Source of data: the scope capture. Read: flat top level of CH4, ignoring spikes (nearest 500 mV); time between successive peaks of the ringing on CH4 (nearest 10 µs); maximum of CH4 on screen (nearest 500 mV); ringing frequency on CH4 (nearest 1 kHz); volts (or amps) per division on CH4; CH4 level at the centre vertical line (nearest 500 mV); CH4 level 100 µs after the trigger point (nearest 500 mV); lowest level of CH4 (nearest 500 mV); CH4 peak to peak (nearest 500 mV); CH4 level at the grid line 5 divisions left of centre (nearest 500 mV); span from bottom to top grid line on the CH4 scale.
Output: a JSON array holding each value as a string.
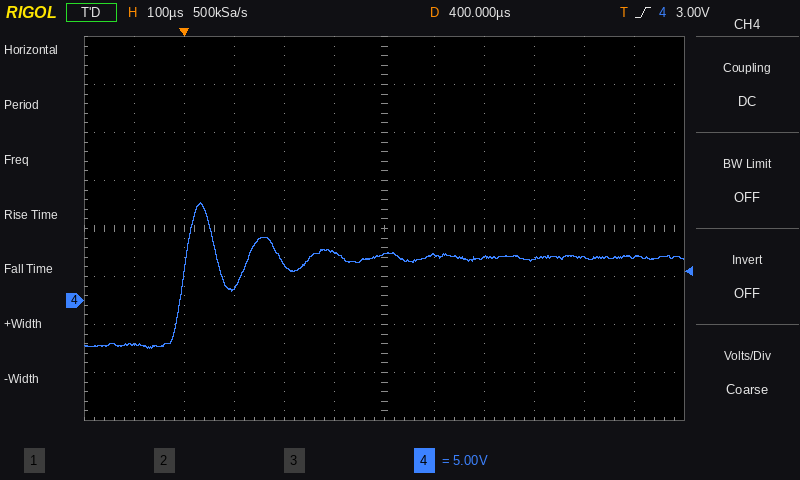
["4.5 V", "130 µs", "10.0 V", "8 kHz", "5 V", "5.0 V", "1.5 V", "-5.0 V", "15.0 V", "-4.5 V", "40 V"]
